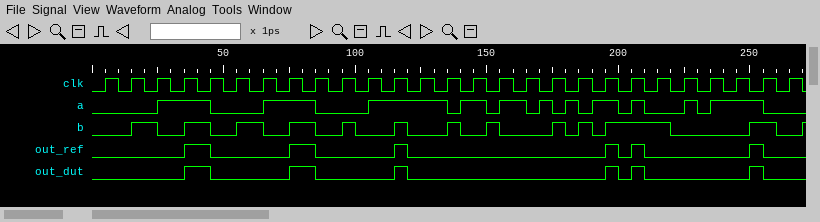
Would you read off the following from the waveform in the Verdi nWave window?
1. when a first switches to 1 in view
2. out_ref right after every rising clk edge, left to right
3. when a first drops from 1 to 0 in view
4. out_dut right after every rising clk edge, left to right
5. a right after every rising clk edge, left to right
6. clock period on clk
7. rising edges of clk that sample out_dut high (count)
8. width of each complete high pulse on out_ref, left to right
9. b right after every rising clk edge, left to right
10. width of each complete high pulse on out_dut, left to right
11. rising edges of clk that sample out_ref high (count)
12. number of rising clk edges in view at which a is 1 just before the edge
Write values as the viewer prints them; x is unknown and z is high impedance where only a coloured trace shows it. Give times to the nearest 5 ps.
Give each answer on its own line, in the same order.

25 ps
0 0 0 1 0 0 0 1 0 0 0 1 0 0 0 0 0 0 0 1 1 0 0 0 0 0 0
45 ps
0 0 0 1 0 0 0 1 0 0 0 1 0 0 0 0 0 0 0 1 1 0 0 0 0 0 0
0 0 1 1 0 0 1 1 0 0 1 1 1 0 1 1 0 0 0 1 1 0 1 1 1 0 0
10 ps
3
10 ps, 10 ps, 5 ps, 5 ps, 5 ps, 5 ps
0 1 0 1 0 1 0 1 0 1 0 1 0 1 0 0 0 1 1 1 1 1 0 0 0 1 0
10 ps, 10 ps, 5 ps, 5 ps, 5 ps, 5 ps
3
14
